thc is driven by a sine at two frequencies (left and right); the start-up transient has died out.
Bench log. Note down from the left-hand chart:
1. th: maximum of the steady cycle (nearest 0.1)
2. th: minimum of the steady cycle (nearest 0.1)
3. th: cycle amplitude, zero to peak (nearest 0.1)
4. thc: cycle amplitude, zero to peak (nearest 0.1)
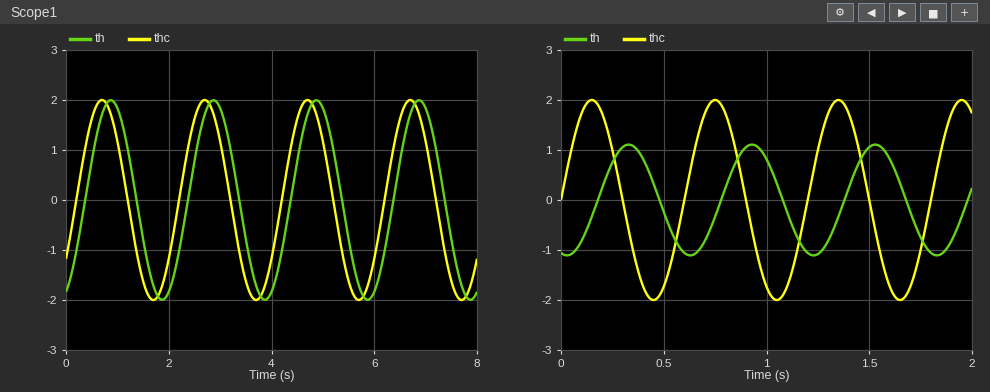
2.0
-2.0
2.0
2.0
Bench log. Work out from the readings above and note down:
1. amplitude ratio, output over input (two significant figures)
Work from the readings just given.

1.0
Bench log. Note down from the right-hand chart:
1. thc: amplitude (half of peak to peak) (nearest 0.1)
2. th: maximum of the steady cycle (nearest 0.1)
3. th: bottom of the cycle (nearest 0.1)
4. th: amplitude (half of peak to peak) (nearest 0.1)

2.0
1.1
-1.1
1.1
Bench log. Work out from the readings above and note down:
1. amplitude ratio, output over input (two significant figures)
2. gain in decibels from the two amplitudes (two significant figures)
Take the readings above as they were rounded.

0.55
-5.2 dB
